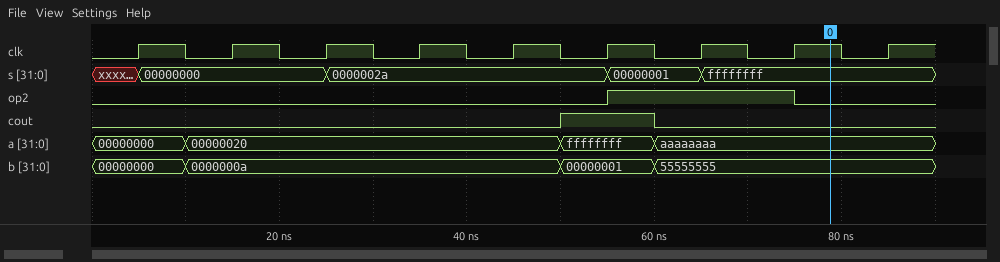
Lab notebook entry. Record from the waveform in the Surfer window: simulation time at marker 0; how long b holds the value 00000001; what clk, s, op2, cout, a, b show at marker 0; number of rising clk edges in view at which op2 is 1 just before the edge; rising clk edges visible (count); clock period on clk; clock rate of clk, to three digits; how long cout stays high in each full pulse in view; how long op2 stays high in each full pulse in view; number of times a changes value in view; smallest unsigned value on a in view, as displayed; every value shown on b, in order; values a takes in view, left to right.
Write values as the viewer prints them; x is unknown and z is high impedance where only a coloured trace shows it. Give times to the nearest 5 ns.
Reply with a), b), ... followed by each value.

a) 80 ns
b) 10 ns
c) clk=1, s=ffffffff, op2=0, cout=0, a=aaaaaaaa, b=55555555
d) 2
e) 9
f) 10 ns
g) 100 MHz
h) 10 ns
i) 20 ns
j) 3
k) 00000000
l) 00000000, 0000000a, 00000001, 55555555
m) 00000000, 00000020, ffffffff, aaaaaaaa
